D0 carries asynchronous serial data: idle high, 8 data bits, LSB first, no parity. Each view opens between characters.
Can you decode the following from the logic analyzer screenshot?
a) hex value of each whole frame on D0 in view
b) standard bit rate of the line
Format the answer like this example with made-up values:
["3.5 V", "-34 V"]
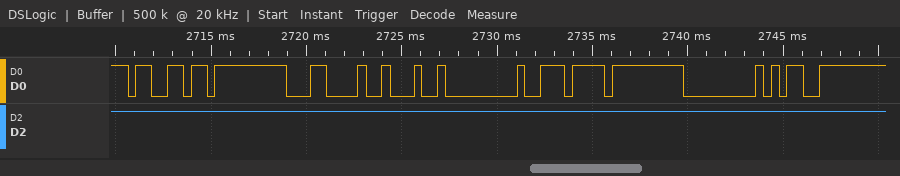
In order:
["B3, FF, 0C, 22, 00, EE, FF, 00, CD", "2400 baud"]
